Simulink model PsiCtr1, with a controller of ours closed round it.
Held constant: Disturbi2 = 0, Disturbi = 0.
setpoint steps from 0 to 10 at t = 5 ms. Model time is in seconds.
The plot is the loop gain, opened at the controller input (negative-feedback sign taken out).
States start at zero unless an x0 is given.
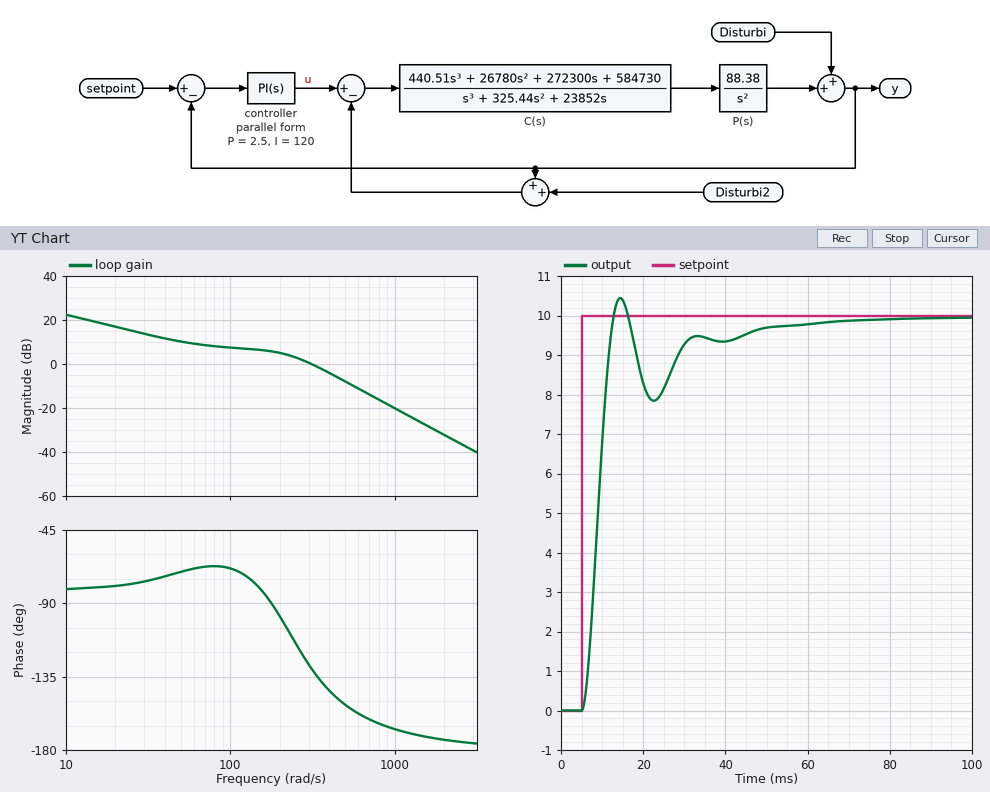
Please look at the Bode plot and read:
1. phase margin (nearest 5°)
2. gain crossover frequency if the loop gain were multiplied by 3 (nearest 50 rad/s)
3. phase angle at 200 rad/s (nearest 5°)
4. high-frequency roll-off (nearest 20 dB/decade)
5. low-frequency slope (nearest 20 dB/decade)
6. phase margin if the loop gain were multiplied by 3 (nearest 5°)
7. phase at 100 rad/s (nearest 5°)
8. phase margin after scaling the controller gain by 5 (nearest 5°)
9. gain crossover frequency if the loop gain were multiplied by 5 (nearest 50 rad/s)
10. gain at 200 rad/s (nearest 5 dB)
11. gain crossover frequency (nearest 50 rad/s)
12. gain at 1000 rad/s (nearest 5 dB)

50°
550 rad/s
-100°
-40 dB/decade
-20 dB/decade
25°
-70°
20°
700 rad/s
5 dB
300 rad/s
-20 dB
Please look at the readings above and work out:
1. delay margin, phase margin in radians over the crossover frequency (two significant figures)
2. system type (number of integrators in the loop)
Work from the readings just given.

0.0029 s
1
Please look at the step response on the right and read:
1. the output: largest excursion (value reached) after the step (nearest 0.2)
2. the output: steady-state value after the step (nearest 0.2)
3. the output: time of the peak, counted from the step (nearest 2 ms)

10.4
10.0
10 ms
